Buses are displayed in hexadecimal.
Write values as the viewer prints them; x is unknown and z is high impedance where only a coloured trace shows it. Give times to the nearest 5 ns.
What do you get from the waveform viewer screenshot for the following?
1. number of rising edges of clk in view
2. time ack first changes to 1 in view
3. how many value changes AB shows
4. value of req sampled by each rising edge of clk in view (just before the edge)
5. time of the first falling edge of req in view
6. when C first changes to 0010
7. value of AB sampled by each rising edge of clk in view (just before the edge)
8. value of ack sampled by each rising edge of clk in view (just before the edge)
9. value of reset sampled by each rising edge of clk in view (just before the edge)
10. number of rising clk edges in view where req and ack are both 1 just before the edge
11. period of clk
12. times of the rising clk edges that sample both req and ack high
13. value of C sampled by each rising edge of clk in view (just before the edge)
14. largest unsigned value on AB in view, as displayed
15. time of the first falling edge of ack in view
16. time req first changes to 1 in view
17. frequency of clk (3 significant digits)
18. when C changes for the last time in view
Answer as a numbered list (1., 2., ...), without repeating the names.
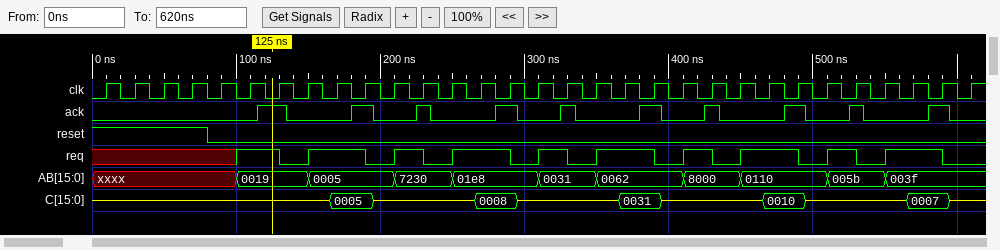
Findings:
1. 31
2. 115 ns
3. 10
4. x x x x x 1 1 0 1 1 0 1 0 1 1 0 1 0 1 1 0 1 0 1 1 0 1 0 1 1 0
5. 130 ns
6. 465 ns
7. xxxx, xxxx, xxxx, xxxx, xxxx, 0019, 0019, 0019, 0005, 0005, 0005, 7230, 7230, 01e8, 01e8, 01e8, 0031, 0031, 0062, 0062, 0062, 8000, 8000, 0110, 0110, 0110, 005b, 005b, 003f, 003f, 003f
8. 0 0 0 0 0 0 1 0 0 1 0 1 0 0 1 0 1 0 0 1 0 1 0 0 1 0 1 0 0 1 0
9. 1 1 1 1 0 0 0 0 0 0 0 0 0 0 0 0 0 0 0 0 0 0 0 0 0 0 0 0 0 0 0
10. 10
11. 20 ns
12. 130 ns, 190 ns, 230 ns, 290 ns, 330 ns, 390 ns, 430 ns, 490 ns, 530 ns, 590 ns
13. z, z, z, z, z, z, z, z, 0005, 0005, z, z, z, 0008, 0008, z, z, z, 0031, 0031, z, z, z, 0010, 0010, z, z, z, 0007, 0007, z
14. 8000
15. 135 ns
16. 100 ns
17. 50.0 MHz
18. 595 ns
